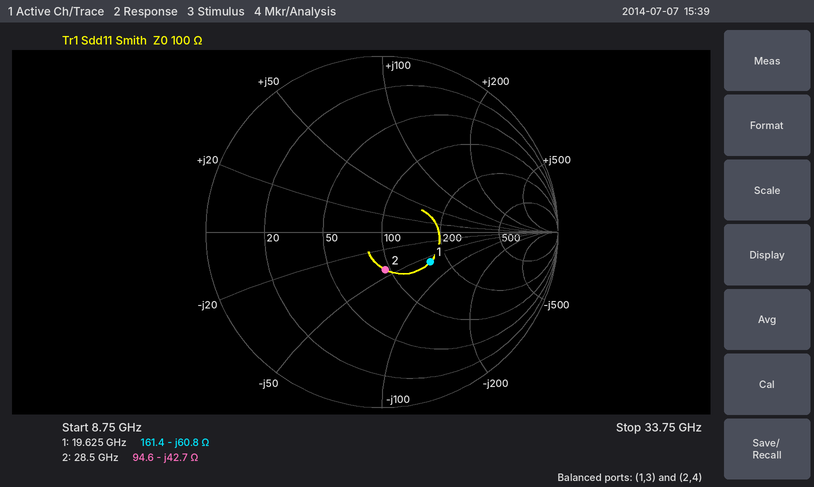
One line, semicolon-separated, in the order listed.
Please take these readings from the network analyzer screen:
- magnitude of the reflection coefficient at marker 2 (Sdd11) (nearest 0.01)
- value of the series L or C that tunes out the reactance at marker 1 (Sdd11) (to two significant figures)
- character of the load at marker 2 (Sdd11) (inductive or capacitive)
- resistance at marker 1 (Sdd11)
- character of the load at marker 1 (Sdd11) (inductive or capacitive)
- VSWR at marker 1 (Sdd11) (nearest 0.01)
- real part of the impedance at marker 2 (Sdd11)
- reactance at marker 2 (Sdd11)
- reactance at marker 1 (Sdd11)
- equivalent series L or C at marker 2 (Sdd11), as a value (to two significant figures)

0.22; 490 pH; capacitive; 161.4 Ω; capacitive; 1.95; 94.6 Ω; -42.7 Ω; -60.8 Ω; 130 fF
